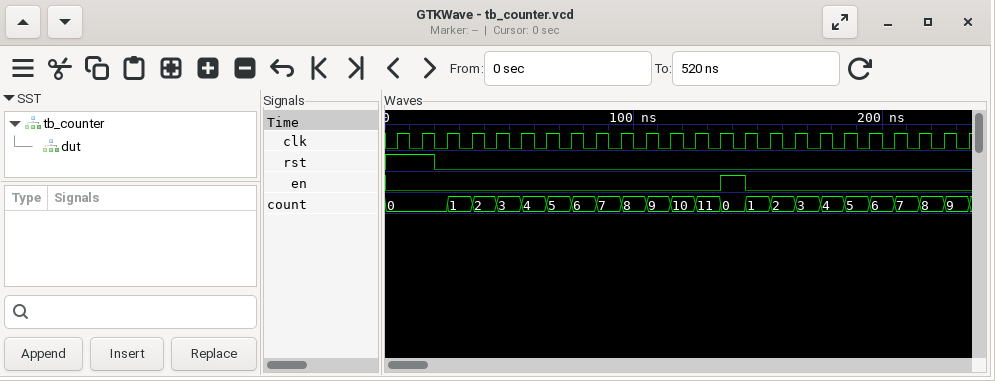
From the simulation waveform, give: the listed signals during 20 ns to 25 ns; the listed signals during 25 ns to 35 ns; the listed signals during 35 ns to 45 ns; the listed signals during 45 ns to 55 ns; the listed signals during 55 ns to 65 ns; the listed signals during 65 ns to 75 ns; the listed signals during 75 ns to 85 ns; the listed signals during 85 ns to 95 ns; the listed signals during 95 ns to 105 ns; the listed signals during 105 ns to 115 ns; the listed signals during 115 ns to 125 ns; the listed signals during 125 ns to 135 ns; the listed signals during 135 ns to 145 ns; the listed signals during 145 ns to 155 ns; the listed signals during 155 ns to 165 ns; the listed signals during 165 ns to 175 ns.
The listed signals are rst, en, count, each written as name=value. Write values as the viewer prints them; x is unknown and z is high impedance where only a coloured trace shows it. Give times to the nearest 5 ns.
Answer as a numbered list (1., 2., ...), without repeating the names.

1. rst=0, en=0, count=0
2. rst=0, en=0, count=1
3. rst=0, en=0, count=2
4. rst=0, en=0, count=3
5. rst=0, en=0, count=4
6. rst=0, en=0, count=5
7. rst=0, en=0, count=6
8. rst=0, en=0, count=7
9. rst=0, en=0, count=8
10. rst=0, en=0, count=9
11. rst=0, en=0, count=10
12. rst=0, en=0, count=11
13. rst=0, en=1, count=0
14. rst=0, en=0, count=1
15. rst=0, en=0, count=2
16. rst=0, en=0, count=3
